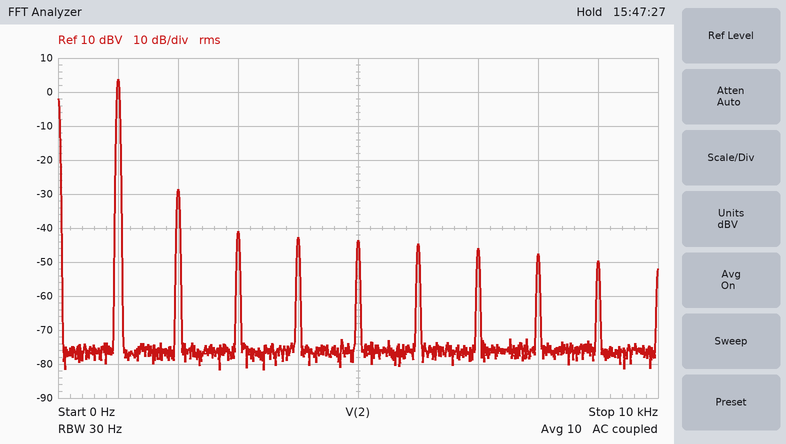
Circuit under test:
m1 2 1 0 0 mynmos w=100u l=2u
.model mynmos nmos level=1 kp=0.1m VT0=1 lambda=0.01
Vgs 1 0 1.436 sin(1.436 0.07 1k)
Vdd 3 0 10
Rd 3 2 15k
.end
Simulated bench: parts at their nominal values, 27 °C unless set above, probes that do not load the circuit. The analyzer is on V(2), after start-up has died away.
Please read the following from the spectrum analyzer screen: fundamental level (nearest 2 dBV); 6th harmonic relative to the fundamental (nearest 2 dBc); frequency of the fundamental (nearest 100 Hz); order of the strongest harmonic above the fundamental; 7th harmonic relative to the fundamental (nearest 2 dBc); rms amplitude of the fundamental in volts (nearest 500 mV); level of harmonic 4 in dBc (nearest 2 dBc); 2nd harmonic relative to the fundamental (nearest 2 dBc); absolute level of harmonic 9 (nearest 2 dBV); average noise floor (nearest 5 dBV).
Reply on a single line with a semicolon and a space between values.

4 dBV; -48 dBc; 1.0 kHz; 2; -50 dBc; 1.5 V; -46 dBc; -32 dBc; -50 dBV; -75 dBV
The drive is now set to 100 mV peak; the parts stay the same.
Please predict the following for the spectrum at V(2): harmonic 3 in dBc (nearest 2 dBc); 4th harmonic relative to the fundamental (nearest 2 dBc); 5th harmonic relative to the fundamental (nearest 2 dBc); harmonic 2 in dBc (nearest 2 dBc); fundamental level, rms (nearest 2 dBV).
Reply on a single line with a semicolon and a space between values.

-24 dBc; -30 dBc; -40 dBc; -26 dBc; 6 dBV
